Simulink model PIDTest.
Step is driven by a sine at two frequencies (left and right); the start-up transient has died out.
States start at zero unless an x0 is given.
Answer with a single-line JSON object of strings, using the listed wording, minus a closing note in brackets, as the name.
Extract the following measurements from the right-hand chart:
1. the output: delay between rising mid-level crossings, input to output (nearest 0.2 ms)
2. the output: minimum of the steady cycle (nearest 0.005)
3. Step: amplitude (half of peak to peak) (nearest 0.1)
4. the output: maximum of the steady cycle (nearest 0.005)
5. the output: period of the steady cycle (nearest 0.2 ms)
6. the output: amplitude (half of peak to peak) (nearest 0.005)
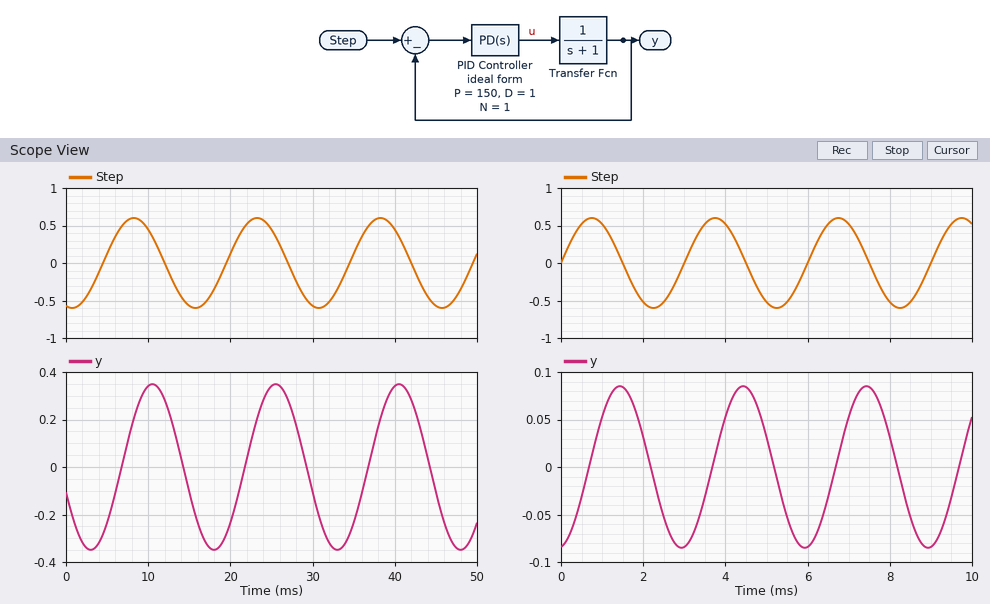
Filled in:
{"the output: delay between rising mid-level crossings, input to output": "0.6 ms", "the output: minimum of the steady cycle": "-0.085", "Step: amplitude (half of peak to peak)": "0.6", "the output: maximum of the steady cycle": "0.085", "the output: period of the steady cycle": "3.0 ms", "the output: amplitude (half of peak to peak)": "0.085"}
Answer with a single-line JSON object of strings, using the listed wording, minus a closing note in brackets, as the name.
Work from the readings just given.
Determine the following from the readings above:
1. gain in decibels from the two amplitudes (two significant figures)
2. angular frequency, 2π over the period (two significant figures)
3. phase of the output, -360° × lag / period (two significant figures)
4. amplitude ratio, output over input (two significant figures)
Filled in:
{"gain in decibels from the two amplitudes": "-17 dB", "angular frequency, 2π over the period": "2.1 rad/ms", "phase of the output, -360° × lag / period": "-72°", "amplitude ratio, output over input": "0.14"}
